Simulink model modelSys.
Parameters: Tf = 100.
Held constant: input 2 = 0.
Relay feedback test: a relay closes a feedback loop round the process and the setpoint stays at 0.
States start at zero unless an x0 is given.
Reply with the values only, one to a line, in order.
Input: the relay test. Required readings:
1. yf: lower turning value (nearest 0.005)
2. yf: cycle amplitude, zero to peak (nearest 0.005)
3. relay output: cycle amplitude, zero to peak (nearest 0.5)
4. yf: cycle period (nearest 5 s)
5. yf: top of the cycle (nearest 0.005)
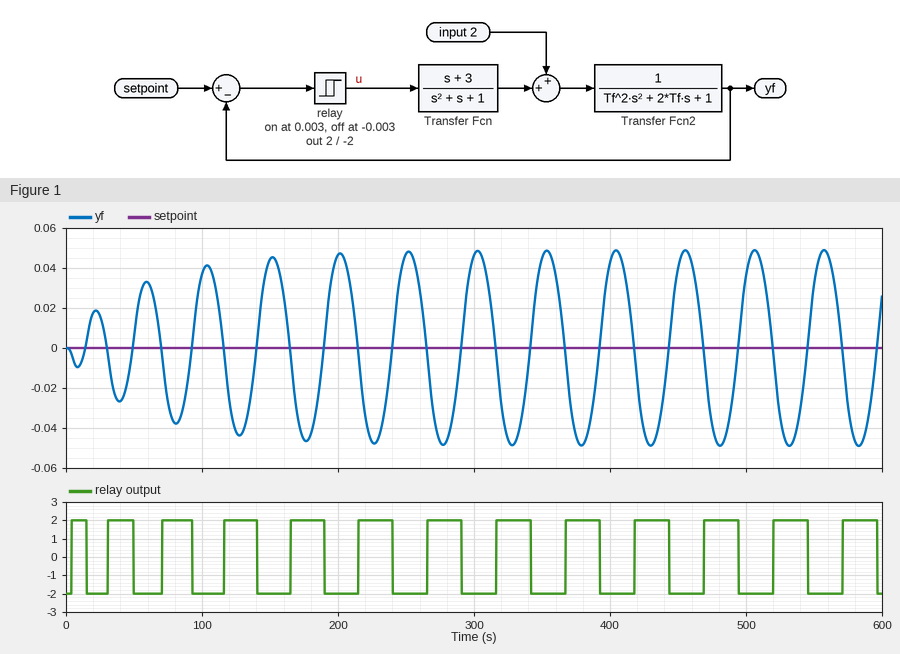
-0.050
0.050
2.0
50 s
0.050
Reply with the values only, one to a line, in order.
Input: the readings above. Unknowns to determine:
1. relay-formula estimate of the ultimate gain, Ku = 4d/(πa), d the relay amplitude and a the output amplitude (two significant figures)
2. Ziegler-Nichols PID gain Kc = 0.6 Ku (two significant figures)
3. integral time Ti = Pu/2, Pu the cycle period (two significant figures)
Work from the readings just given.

51
31
25 s
